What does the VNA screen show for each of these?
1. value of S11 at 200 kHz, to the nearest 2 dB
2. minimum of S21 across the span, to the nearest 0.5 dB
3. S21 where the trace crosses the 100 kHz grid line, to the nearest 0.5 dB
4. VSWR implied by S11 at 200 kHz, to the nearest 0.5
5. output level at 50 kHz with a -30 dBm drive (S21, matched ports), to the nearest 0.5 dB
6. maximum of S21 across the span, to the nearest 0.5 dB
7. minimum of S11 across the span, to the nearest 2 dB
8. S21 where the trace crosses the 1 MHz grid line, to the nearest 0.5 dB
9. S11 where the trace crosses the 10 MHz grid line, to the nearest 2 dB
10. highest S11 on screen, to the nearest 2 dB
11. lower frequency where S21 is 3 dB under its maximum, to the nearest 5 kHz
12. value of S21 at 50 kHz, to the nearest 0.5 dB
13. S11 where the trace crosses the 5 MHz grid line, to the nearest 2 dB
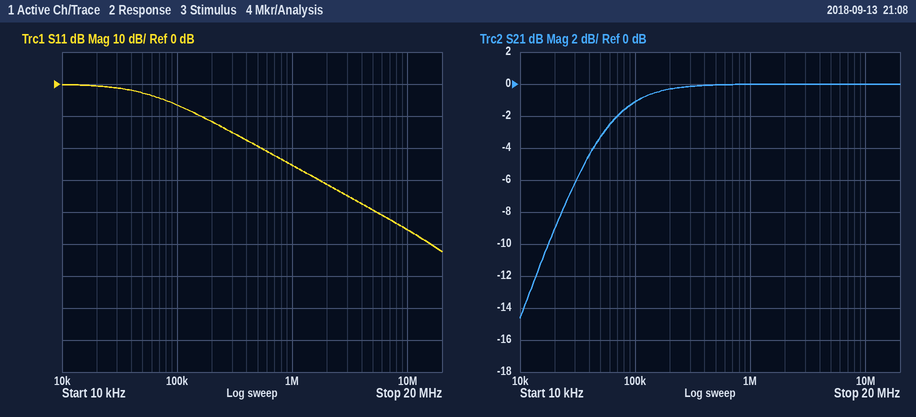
-12 dB
-14.5 dB
-1.0 dB
1.5
-33.5 dBm
0.0 dB
-52 dB
0.0 dB
-46 dB
0 dB
55 kHz
-3.5 dB
-40 dB
